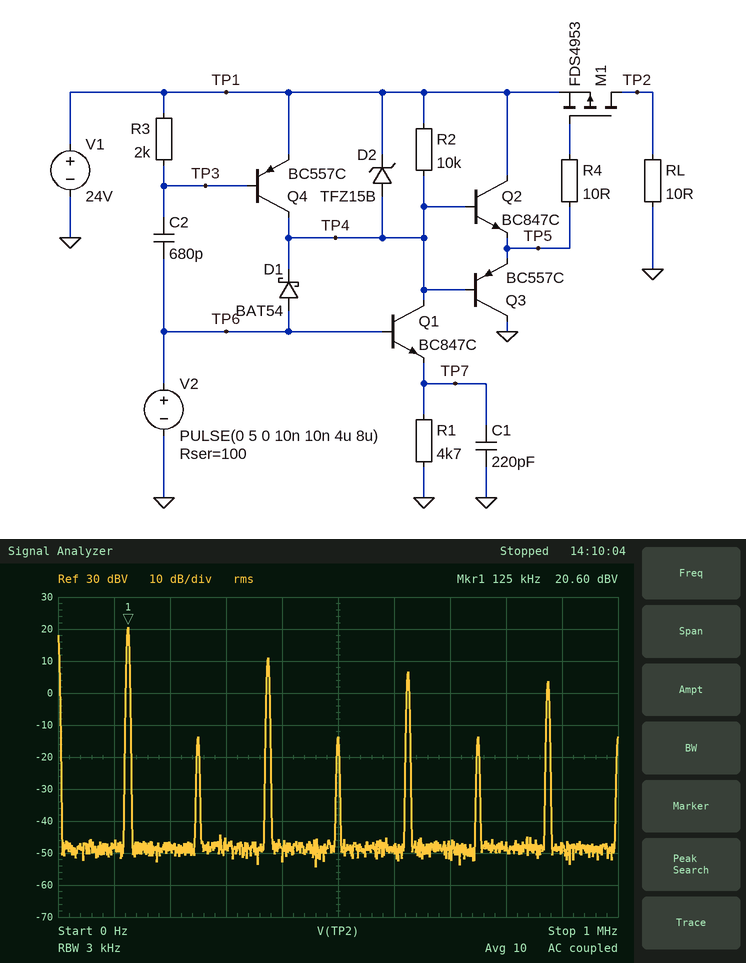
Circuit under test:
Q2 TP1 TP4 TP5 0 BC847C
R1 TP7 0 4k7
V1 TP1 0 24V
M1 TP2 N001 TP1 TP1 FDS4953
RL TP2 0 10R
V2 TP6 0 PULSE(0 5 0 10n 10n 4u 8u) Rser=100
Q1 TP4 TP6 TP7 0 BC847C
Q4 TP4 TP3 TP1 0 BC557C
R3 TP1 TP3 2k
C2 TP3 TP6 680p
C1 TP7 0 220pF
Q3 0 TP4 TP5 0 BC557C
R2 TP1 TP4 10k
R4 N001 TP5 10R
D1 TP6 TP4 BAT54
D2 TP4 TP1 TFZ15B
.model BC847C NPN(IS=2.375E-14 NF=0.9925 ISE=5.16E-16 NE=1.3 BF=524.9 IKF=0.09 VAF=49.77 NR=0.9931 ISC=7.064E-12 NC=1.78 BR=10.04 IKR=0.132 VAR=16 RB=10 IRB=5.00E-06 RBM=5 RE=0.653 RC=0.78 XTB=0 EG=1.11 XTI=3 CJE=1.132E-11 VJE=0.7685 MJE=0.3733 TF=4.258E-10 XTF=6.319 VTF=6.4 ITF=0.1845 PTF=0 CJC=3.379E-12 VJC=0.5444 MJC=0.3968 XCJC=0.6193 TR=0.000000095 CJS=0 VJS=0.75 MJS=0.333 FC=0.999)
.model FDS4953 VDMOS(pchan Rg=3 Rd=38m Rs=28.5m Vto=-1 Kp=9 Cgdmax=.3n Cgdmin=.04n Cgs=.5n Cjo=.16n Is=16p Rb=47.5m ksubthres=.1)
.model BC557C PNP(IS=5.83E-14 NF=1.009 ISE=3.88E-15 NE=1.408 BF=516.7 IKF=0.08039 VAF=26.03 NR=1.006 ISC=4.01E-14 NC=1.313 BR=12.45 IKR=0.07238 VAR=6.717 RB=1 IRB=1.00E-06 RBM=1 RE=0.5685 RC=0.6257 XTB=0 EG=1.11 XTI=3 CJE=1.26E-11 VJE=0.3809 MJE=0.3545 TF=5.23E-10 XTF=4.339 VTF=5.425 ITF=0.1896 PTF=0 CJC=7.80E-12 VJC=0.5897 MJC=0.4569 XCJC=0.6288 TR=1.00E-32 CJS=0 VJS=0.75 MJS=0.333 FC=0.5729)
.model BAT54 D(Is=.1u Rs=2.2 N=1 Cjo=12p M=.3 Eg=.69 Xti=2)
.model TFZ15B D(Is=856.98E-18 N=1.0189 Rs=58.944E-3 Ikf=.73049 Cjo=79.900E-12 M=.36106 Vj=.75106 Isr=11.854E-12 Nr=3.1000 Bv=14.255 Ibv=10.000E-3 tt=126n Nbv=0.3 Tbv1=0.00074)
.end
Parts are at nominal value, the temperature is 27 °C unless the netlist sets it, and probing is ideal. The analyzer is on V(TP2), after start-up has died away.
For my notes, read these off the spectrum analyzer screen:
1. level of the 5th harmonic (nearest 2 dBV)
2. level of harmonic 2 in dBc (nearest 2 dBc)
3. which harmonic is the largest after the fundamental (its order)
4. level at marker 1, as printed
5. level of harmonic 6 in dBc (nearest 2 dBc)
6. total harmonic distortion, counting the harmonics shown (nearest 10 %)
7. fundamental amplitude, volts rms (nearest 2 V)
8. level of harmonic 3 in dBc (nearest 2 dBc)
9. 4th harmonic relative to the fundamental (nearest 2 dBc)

6 dBV
-34 dBc
3
20.60 dBV
-34 dBc
40 %
10 V
-10 dBc
-34 dBc
